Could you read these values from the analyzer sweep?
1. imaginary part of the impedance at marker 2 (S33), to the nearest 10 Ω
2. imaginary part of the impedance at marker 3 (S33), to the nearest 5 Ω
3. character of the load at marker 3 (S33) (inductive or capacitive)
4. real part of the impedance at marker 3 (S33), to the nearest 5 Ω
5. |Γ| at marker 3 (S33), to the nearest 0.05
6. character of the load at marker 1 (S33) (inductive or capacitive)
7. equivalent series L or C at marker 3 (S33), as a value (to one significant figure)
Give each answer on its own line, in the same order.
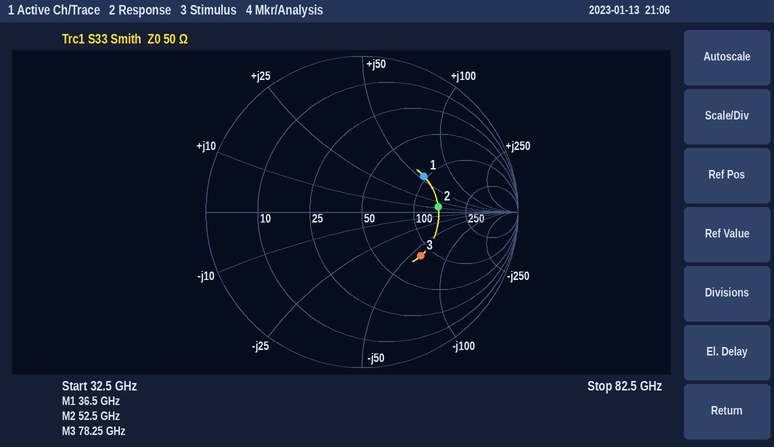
+10 Ω
-60 Ω
capacitive
85 Ω
0.45
inductive
30 fF
